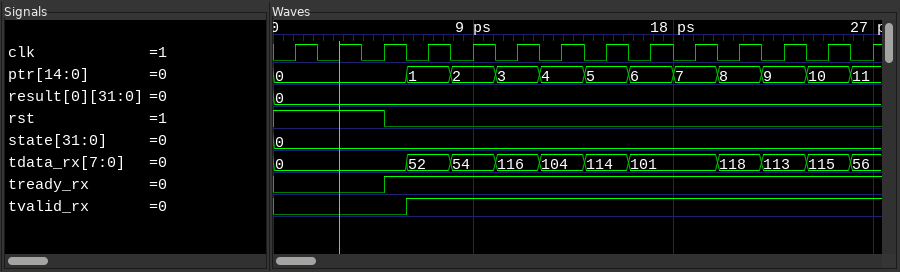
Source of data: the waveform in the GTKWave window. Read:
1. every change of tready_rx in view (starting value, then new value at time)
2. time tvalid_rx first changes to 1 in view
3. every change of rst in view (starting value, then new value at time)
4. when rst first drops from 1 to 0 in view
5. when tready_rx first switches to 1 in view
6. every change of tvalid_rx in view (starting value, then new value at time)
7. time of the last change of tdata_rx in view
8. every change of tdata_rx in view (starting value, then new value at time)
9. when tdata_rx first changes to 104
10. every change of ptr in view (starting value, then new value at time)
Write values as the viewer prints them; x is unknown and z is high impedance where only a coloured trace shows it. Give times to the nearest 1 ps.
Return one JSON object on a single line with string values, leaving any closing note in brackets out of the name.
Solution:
{"every change of tready_rx in view": "0, 1 at 5 ps", "time tvalid_rx first changes to 1 in view": "6 ps", "every change of rst in view": "1, 0 at 5 ps", "when rst first drops from 1 to 0 in view": "5 ps", "when tready_rx first switches to 1 in view": "5 ps", "every change of tvalid_rx in view": "0, 1 at 6 ps", "time of the last change of tdata_rx in view": "26 ps", "every change of tdata_rx in view": "0, 52 at 6 ps, 54 at 8 ps, 116 at 10 ps, 104 at 12 ps, 114 at 14 ps, 101 at 16 ps, 118 at 20 ps, 113 at 22 ps, 115 at 24 ps, 56 at 26 ps", "when tdata_rx first changes to 104": "12 ps", "every change of ptr in view": "0, 1 at 6 ps, 2 at 8 ps, 3 at 10 ps, 4 at 12 ps, 5 at 14 ps, 6 at 16 ps, 7 at 18 ps, 8 at 20 ps, 9 at 22 ps, 10 at 24 ps, 11 at 26 ps"}
